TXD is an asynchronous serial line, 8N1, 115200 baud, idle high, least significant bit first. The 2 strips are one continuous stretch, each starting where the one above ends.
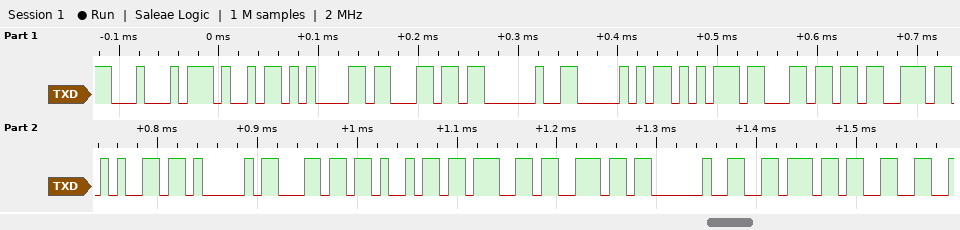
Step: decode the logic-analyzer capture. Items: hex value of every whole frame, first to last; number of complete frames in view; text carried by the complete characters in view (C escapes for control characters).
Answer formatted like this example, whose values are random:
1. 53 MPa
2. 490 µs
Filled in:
1. 44 69 61 6C 20 50 75 6C 73 65 41 6C 69 67 6E 20 76 33
2. 18
3. "Dial PulseAlign v3"
